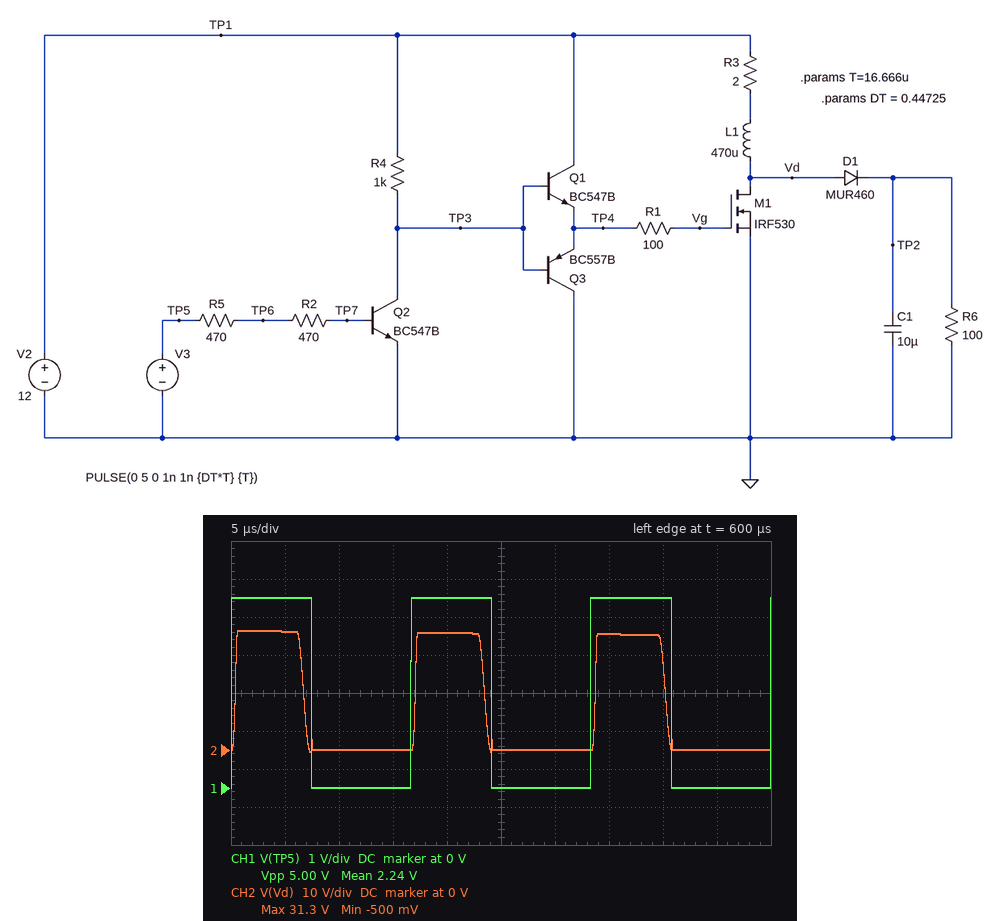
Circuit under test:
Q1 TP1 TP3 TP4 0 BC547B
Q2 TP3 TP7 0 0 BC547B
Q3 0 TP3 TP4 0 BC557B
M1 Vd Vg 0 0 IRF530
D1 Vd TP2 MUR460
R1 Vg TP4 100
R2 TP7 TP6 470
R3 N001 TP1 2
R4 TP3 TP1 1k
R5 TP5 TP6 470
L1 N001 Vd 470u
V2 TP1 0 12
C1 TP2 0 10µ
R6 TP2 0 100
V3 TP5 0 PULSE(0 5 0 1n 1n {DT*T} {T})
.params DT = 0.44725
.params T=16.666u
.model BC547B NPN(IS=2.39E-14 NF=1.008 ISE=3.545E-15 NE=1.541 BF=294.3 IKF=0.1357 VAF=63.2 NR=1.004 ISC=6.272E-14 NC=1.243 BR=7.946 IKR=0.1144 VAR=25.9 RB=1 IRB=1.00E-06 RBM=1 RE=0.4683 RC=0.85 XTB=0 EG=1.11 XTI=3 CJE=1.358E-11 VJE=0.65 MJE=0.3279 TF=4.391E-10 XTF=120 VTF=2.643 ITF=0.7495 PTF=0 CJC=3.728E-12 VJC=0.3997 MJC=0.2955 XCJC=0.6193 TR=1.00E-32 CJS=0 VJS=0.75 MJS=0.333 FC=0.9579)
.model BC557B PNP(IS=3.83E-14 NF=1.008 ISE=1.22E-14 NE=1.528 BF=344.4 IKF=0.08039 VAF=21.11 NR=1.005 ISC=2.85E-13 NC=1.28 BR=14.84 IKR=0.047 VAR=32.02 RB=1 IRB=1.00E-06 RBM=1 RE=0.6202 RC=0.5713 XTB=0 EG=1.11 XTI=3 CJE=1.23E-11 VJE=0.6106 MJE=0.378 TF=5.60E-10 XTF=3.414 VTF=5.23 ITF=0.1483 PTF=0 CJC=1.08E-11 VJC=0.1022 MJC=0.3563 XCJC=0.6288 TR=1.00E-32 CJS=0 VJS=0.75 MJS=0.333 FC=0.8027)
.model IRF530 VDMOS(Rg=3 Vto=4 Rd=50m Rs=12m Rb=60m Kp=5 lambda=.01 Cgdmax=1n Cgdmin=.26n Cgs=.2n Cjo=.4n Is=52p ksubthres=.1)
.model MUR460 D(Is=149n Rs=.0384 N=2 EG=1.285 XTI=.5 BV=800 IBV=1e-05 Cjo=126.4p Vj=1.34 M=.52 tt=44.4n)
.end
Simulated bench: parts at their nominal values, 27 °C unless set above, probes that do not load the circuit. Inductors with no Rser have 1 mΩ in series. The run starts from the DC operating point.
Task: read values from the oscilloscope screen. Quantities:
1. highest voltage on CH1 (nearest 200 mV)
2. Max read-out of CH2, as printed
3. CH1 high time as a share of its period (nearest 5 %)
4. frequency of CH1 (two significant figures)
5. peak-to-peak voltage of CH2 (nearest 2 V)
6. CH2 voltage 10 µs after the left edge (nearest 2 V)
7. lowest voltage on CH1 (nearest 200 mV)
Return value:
5.0 V
31.3 V
45 %
60 kHz
32 V
0 V
0 V
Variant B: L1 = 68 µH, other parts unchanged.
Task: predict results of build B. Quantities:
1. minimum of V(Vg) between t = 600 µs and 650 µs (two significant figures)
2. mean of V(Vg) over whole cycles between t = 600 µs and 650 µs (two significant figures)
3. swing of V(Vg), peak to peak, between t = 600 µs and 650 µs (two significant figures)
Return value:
-2.7 V
6.5 V
14 V
